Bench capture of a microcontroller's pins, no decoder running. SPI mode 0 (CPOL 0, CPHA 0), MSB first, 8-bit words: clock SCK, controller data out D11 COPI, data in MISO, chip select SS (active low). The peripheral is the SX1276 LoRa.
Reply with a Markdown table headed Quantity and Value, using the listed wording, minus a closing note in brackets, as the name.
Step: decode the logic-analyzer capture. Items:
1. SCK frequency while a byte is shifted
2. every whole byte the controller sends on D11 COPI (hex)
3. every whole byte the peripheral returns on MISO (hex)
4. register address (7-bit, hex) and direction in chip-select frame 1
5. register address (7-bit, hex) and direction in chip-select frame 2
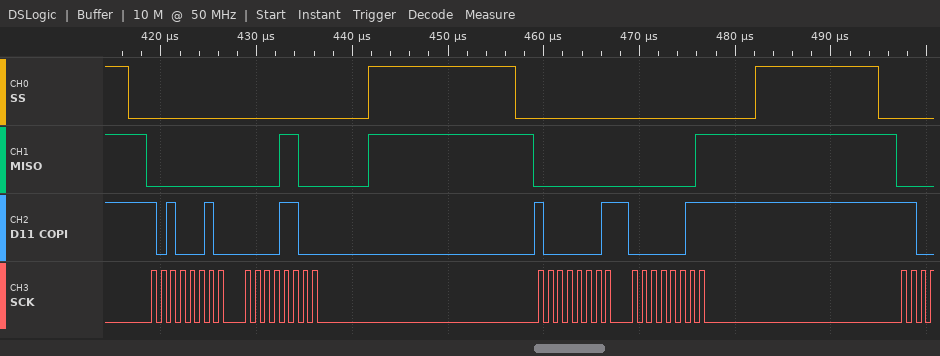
| Quantity | Value |
|---|---|
| SCK frequency while a byte is shifted | 1 MHz |
| every whole byte the controller sends on D11 COPI | A2 0C 81 03 |
| every whole byte the peripheral returns on MISO | 00 0C 00 01 |
| register address (7-bit, hex) and direction in chip-select frame 1 | 0x22 write |
| register address (7-bit, hex) and direction in chip-select frame 2 | 0x01 write |
